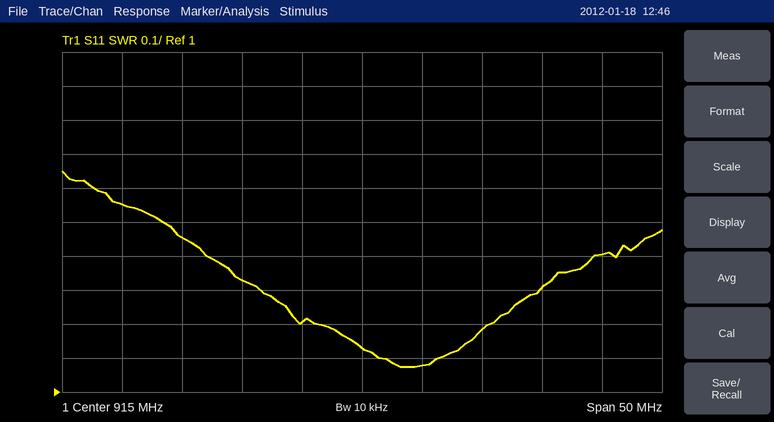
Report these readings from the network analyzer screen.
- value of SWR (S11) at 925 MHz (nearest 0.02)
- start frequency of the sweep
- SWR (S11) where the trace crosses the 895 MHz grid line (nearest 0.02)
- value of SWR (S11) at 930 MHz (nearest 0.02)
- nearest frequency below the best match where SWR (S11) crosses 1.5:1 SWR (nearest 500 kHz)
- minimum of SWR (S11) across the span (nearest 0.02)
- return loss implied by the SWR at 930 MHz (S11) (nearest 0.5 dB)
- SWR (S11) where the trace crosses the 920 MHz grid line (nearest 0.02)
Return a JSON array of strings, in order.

["1.18", "890 MHz", "1.56", "1.30", "898.5 MHz", "1.08", "17.5 dB", "1.08"]
